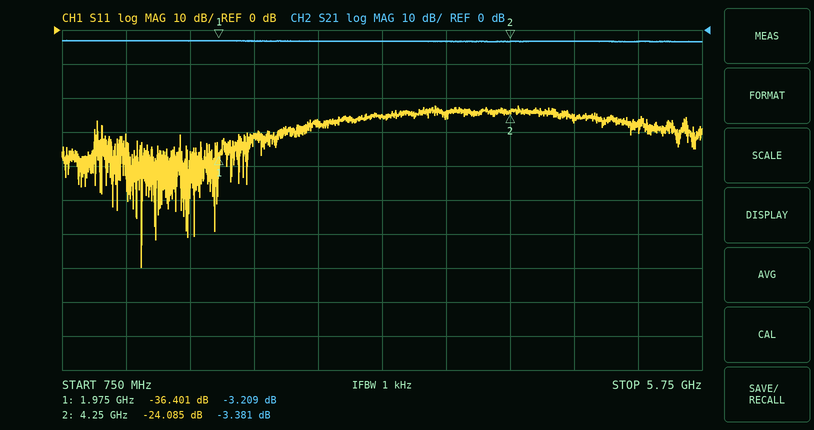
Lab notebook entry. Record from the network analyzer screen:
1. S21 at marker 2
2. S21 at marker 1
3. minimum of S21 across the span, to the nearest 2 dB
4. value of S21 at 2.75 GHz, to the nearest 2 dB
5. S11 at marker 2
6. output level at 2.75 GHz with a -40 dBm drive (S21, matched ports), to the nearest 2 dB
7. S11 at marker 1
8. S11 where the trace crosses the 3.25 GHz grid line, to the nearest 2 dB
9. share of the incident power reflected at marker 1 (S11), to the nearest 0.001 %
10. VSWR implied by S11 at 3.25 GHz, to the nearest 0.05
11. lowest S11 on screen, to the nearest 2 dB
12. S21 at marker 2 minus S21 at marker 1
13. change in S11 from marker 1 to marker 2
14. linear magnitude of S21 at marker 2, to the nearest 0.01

-3.381 dB
-3.209 dB
-4 dB
-4 dB
-24.085 dB
-44 dBm
-36.401 dB
-26 dB
0.023 %
1.10
-70 dB
-0.172 dB
12.316 dB
0.68
